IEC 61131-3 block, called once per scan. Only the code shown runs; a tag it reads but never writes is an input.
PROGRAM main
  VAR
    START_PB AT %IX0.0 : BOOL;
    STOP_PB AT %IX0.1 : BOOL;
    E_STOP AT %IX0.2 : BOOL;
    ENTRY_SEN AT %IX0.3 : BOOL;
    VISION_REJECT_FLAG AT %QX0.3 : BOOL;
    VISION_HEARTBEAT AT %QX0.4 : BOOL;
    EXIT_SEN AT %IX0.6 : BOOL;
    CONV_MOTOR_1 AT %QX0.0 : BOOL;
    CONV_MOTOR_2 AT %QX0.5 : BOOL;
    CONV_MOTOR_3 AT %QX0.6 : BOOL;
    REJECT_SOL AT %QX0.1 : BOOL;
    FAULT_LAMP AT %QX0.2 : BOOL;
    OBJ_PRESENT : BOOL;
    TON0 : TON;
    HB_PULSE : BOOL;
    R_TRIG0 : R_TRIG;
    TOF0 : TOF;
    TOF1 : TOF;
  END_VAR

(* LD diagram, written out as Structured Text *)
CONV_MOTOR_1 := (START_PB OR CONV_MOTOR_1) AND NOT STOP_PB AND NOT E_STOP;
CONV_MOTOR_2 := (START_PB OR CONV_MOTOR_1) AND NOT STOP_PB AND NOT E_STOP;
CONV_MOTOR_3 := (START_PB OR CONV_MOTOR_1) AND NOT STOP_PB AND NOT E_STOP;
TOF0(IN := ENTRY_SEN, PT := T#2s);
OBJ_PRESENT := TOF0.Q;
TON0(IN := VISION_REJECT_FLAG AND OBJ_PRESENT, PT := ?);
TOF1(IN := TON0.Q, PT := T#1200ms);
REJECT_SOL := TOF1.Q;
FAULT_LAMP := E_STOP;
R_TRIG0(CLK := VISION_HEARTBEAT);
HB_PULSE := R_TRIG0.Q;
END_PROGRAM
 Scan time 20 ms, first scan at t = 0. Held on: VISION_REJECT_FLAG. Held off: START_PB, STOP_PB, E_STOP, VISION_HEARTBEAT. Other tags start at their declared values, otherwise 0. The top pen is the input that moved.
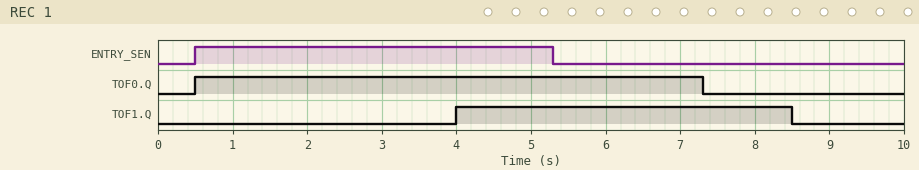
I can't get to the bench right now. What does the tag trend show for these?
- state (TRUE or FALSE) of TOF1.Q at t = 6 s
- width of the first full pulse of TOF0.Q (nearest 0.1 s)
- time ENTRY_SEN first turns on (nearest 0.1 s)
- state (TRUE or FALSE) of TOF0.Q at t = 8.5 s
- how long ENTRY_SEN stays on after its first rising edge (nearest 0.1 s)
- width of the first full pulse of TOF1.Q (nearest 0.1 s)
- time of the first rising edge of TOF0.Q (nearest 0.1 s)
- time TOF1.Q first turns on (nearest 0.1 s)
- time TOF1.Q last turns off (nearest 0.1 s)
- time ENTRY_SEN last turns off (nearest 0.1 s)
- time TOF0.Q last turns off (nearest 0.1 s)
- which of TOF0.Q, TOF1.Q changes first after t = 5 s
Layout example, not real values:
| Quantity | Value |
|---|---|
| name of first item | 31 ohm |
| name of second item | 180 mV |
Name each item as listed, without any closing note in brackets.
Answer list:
| Quantity | Value |
|---|---|
| state (TRUE or FALSE) of TOF1.Q at t = 6 s | TRUE |
| width of the first full pulse of TOF0.Q | 6.8 s |
| time ENTRY_SEN first turns on | 0.5 s |
| state (TRUE or FALSE) of TOF0.Q at t = 8.5 s | FALSE |
| how long ENTRY_SEN stays on after its first rising edge | 4.8 s |
| width of the first full pulse of TOF1.Q | 4.5 s |
| time of the first rising edge of TOF0.Q | 0.5 s |
| time TOF1.Q first turns on | 4.0 s |
| time TOF1.Q last turns off | 8.5 s |
| time ENTRY_SEN last turns off | 5.3 s |
| time TOF0.Q last turns off | 7.3 s |
| which of TOF0.Q, TOF1.Q changes first after t = 5 s | TOF0.Q |
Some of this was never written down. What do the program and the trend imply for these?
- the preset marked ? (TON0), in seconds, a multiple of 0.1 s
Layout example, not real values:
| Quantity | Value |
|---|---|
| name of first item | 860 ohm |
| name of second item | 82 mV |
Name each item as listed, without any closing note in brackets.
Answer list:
| Quantity | Value |
|---|---|
| the preset marked ? (TON0), in seconds, a multiple of 0.1 s | 3.5 s |
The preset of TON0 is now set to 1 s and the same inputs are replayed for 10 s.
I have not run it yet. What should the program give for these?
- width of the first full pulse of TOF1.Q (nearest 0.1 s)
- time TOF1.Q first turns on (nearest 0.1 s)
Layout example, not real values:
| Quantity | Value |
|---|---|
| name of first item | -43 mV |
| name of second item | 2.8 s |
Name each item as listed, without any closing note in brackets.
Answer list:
| Quantity | Value |
|---|---|
| width of the first full pulse of TOF1.Q | 7.0 s |
| time TOF1.Q first turns on | 1.5 s |
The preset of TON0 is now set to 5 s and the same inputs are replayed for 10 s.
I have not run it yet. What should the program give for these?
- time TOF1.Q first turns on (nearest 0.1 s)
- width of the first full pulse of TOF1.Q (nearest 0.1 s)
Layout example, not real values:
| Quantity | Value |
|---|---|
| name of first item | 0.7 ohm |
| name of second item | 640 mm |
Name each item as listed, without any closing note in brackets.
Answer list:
| Quantity | Value |
|---|---|
| time TOF1.Q first turns on | 5.5 s |
| width of the first full pulse of TOF1.Q | 3.0 s |
